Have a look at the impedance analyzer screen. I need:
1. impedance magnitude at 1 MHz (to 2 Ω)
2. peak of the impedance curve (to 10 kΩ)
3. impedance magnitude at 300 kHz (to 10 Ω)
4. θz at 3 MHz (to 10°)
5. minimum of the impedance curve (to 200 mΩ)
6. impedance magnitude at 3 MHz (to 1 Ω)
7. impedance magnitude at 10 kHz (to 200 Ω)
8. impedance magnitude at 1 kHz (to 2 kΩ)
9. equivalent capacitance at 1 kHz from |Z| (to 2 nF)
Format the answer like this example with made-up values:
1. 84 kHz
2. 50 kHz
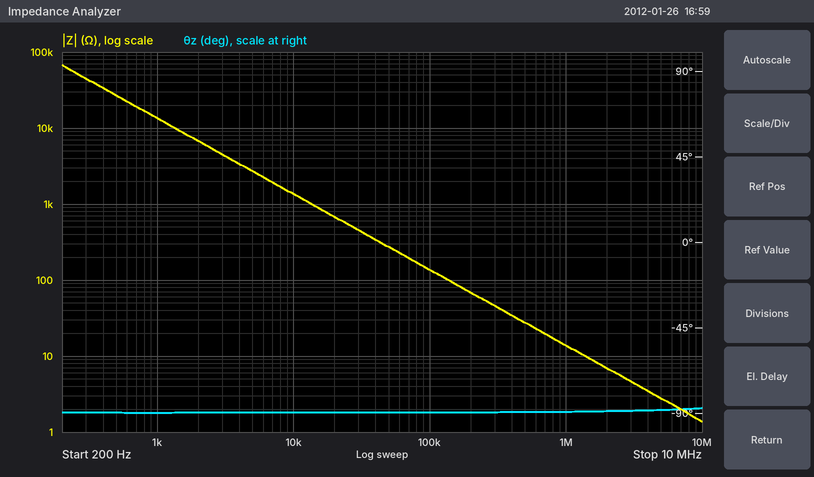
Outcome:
1. 14 Ω
2. 70 kΩ
3. 50 Ω
4. -90°
5. 1.4 Ω
6. 5 Ω
7. 1.4 kΩ
8. 14 kΩ
9. 12 nF
